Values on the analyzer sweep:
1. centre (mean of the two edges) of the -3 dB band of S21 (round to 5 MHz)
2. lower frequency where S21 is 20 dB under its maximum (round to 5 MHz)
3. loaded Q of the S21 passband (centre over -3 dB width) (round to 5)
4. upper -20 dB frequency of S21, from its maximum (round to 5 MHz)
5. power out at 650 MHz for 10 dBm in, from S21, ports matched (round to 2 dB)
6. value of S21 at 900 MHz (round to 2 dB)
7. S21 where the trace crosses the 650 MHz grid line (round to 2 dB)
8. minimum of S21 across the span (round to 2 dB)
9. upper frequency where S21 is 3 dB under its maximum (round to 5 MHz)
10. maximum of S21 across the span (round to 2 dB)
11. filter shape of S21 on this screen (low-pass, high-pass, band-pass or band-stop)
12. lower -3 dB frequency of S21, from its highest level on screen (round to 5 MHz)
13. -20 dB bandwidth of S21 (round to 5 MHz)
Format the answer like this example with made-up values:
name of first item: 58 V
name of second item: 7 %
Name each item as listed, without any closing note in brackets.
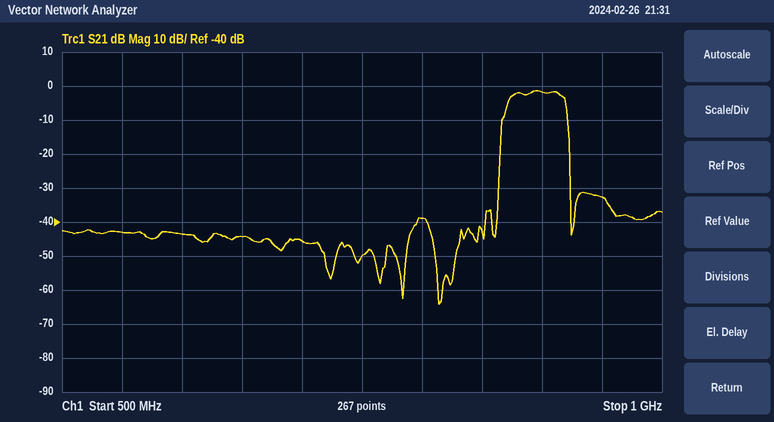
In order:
centre (mean of the two edges) of the -3 dB band of S21: 895 MHz
lower frequency where S21 is 20 dB under its maximum: 865 MHz
loaded Q of the S21 passband (centre over -3 dB width): 20
upper -20 dB frequency of S21, from its maximum: 925 MHz
power out at 650 MHz for 10 dBm in, from S21, ports matched: -34 dBm
value of S21 at 900 MHz: -2 dB
S21 where the trace crosses the 650 MHz grid line: -44 dB
minimum of S21 across the span: -64 dB
upper frequency where S21 is 3 dB under its maximum: 920 MHz
maximum of S21 across the span: -2 dB
filter shape of S21 on this screen: band-pass
lower -3 dB frequency of S21, from its highest level on screen: 870 MHz
-20 dB bandwidth of S21: 60 MHz
